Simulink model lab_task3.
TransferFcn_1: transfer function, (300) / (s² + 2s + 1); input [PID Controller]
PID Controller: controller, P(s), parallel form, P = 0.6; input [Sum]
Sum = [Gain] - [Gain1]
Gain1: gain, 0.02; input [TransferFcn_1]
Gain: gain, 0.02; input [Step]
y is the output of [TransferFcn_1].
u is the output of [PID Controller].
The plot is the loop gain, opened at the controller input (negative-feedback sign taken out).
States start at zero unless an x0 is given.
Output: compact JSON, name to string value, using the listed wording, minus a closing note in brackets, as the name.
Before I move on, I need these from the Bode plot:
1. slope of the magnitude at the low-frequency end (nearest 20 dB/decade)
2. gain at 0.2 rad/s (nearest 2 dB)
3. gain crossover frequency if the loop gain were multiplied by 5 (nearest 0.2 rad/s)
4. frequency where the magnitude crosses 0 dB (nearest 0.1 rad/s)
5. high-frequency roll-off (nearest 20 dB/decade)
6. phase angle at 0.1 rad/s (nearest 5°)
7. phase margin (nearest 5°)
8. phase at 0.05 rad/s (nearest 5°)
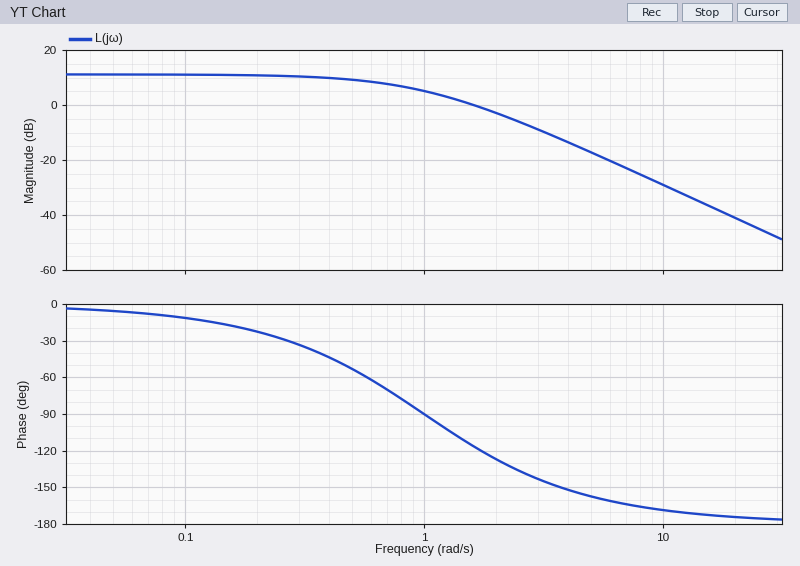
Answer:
{"slope of the magnitude at the low-frequency end": "0 dB/decade", "gain at 0.2 rad/s": "10 dB", "gain crossover frequency if the loop gain were multiplied by 5": "4.2 rad/s", "frequency where the magnitude crosses 0 dB": "1.6 rad/s", "high-frequency roll-off": "-40 dB/decade", "phase angle at 0.1 rad/s": "-10°", "phase margin": "65°", "phase at 0.05 rad/s": "-5°"}
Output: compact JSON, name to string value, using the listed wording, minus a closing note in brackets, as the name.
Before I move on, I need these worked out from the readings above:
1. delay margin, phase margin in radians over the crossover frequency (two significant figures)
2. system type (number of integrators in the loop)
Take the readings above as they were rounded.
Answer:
{"delay margin, phase margin in radians over the crossover frequency": "0.71 s", "system type": "0"}
